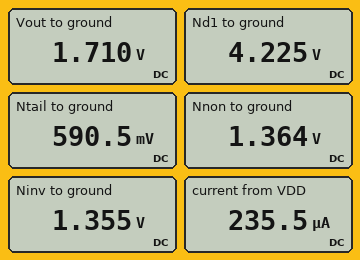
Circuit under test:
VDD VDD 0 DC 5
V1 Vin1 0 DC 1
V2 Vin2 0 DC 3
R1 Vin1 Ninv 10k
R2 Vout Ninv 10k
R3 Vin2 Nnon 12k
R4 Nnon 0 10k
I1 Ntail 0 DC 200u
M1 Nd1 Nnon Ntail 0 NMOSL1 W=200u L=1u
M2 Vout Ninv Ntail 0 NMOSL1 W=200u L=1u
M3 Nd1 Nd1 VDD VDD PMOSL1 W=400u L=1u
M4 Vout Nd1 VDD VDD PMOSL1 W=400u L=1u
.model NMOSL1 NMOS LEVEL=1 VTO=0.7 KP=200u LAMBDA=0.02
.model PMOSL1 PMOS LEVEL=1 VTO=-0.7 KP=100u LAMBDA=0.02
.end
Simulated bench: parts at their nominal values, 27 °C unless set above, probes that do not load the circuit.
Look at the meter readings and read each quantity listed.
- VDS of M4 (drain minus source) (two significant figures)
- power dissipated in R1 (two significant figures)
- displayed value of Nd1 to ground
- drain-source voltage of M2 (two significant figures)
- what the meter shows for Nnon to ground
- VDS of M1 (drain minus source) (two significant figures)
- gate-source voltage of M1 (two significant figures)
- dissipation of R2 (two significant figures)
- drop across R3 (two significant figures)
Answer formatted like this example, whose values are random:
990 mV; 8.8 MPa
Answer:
-3.3 V; 13 µW; 4.225 V; 1.1 V; 1.364 V; 3.6 V; 770 mV; 13 µW; 1.6 V
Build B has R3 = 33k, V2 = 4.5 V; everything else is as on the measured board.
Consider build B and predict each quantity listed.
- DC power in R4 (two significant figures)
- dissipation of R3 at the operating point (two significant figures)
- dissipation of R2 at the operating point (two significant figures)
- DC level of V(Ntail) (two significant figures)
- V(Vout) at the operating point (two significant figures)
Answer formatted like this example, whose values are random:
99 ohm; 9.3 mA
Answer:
110 µW; 360 µW; 240 nW; 280 mV; 1.1 V
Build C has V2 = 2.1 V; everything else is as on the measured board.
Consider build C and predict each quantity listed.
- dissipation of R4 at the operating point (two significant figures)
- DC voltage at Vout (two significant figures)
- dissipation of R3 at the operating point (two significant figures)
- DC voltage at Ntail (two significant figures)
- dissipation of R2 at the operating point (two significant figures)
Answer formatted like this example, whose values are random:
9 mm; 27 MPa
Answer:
91 µW; 920 mV; 110 µW; 190 mV; 160 nW
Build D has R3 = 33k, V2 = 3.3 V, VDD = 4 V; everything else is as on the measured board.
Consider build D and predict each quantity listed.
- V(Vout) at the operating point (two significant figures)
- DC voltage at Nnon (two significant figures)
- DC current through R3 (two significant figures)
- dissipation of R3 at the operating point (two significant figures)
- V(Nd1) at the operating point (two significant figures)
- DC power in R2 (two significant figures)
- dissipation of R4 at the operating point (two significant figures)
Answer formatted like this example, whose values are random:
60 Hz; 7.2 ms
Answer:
560 mV; 770 mV; 77 µA; 190 µW; 3.2 V; 4.9 µW; 59 µW
